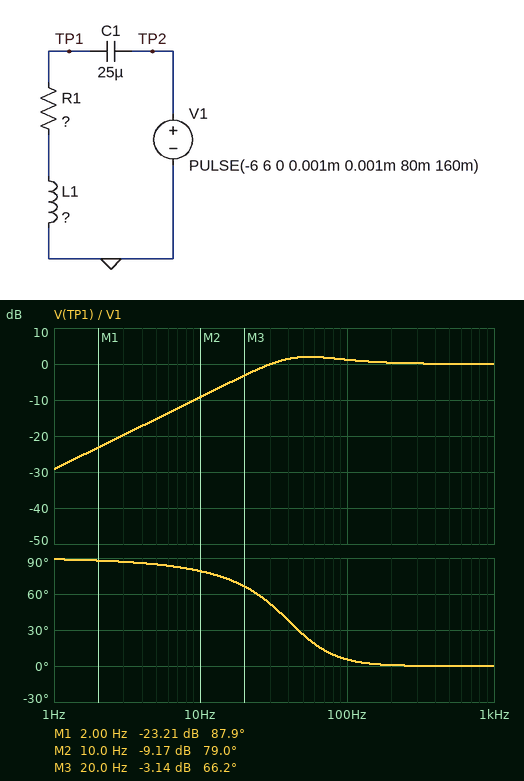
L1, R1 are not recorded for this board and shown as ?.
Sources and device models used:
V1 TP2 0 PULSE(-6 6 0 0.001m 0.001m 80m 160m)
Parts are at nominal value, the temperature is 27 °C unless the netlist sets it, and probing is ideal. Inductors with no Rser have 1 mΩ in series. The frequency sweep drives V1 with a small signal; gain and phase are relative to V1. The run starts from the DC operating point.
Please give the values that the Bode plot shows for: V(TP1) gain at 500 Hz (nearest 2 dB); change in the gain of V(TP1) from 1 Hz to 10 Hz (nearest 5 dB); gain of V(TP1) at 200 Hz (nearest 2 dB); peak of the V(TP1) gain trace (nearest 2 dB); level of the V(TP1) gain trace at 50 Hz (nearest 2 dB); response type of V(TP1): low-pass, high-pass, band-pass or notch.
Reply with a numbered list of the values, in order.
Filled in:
1. 0 dB
2. 20 dB
3. 0 dB
4. 2 dB
5. 2 dB
6. high-pass
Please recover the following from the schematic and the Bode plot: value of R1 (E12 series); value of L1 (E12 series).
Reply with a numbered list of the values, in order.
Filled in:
1. 220 Ω
2. 560 mH
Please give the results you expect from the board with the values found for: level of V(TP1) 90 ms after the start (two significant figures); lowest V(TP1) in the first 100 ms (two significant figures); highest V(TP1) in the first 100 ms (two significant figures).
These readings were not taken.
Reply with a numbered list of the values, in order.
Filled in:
1. -1.4 V
2. -12 V
3. 12 V
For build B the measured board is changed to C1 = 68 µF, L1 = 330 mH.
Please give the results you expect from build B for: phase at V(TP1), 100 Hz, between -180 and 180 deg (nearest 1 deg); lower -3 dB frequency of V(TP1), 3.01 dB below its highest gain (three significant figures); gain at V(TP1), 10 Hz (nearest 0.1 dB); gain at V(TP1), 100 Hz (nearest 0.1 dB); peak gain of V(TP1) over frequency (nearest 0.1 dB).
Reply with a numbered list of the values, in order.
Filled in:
1. 3 deg
2. 10.9 Hz
3. -2.8 dB
4. 0.5 dB
5. 0.6 dB
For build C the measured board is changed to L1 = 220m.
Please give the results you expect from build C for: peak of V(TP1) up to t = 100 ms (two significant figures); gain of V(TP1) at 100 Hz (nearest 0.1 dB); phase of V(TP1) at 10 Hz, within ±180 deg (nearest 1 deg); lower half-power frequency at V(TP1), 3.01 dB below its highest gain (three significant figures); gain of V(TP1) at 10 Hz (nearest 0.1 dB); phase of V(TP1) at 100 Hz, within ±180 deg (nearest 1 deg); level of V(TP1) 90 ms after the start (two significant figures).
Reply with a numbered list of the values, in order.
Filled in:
1. 12 V
2. 1.0 dB
3. 74 deg
4. 29.2 Hz
5. -9.5 dB
6. 13 deg
7. -1.6 V
